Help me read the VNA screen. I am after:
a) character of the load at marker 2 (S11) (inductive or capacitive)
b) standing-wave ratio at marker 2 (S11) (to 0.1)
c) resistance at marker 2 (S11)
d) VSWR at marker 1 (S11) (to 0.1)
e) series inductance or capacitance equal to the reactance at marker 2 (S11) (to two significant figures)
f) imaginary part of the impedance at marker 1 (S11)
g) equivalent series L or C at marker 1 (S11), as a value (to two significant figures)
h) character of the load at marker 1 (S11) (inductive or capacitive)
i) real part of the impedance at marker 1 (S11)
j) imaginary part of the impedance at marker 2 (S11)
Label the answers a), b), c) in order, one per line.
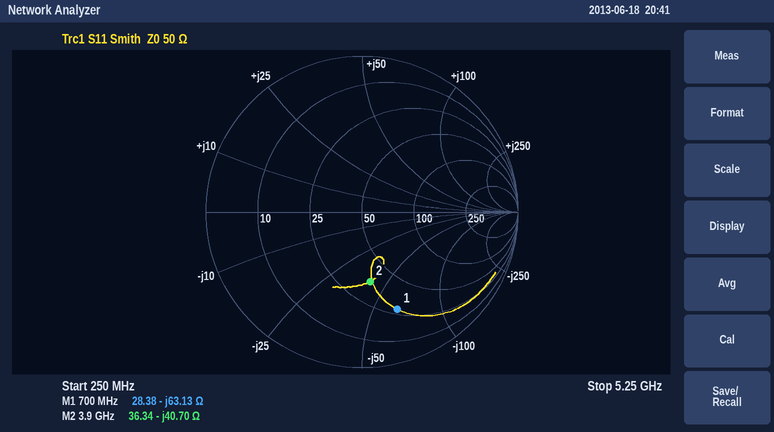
a) capacitive
b) 2.6
c) 36.34 Ω
d) 4.9
e) 1.0 pF
f) -63.13 Ω
g) 3.6 pF
h) capacitive
i) 28.38 Ω
j) -40.70 Ω
